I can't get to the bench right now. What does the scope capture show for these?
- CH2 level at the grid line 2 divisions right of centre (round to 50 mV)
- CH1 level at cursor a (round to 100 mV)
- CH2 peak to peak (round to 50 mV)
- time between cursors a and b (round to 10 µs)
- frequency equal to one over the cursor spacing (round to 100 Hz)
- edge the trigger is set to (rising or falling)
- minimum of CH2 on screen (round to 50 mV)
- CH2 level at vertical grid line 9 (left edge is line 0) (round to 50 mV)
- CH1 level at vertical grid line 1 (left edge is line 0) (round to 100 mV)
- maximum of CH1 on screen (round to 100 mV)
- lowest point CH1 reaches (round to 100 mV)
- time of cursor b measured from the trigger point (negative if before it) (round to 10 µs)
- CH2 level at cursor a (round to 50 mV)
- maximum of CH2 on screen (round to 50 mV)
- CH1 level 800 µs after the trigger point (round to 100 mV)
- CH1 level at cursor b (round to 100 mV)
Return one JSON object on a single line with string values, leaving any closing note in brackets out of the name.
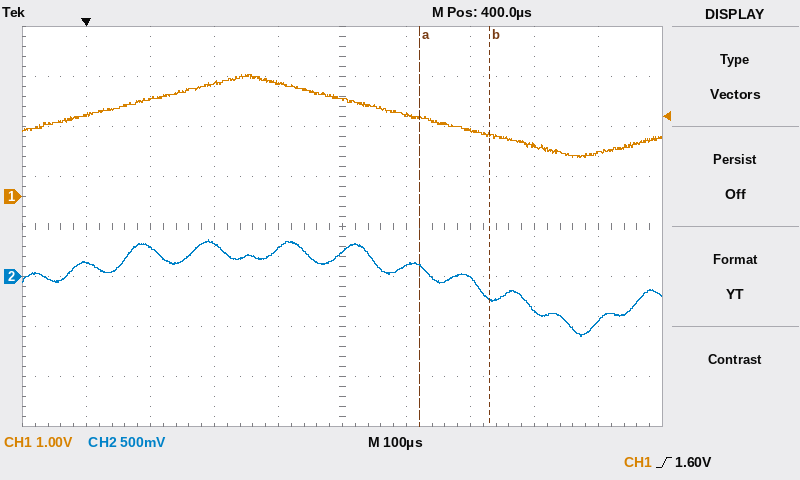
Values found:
{"CH2 level at the grid line 2 divisions right of centre": "0 mV", "CH1 level at cursor a": "1.6 V", "CH2 peak to peak": "950 mV", "time between cursors a and b": "110 µs", "frequency equal to one over the cursor spacing": "9.1 kHz", "edge the trigger is set to": "rising", "minimum of CH2 on screen": "-600 mV", "CH2 level at vertical grid line 9 (left edge is line 0)": "-450 mV", "CH1 level at vertical grid line 1 (left edge is line 0)": "1.6 V", "maximum of CH1 on screen": "2.4 V", "lowest point CH1 reaches": "800 mV", "time of cursor b measured from the trigger point (negative if before it)": "+630 µs", "CH2 level at cursor a": "100 mV", "maximum of CH2 on screen": "350 mV", "CH1 level 800 µs after the trigger point": "900 mV", "CH1 level at cursor b": "1.2 V"}
